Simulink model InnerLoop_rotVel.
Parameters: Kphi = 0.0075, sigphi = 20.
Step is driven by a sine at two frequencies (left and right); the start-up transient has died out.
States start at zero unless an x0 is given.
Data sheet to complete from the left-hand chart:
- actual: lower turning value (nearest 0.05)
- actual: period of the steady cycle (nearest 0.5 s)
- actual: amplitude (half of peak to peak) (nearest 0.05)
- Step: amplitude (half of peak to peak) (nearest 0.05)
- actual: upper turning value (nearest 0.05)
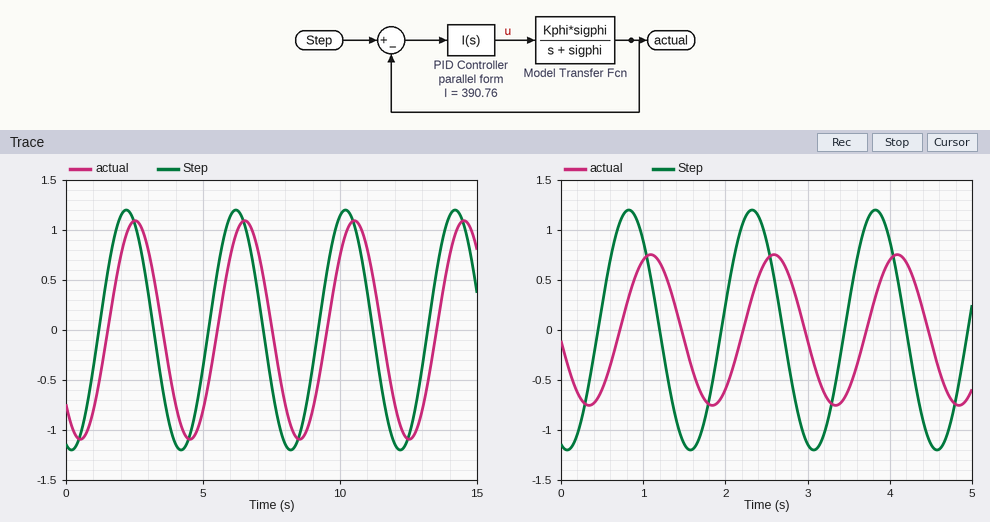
-1.10
4.0 s
1.10
1.20
1.10
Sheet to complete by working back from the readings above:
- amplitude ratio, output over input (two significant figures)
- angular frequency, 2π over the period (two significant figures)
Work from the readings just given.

0.92
1.6 rad/s
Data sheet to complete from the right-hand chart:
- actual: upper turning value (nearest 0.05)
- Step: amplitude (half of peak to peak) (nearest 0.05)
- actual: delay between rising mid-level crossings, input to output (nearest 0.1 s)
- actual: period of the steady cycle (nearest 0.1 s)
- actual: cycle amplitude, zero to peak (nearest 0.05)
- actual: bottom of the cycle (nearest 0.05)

0.75
1.20
0.3 s
1.5 s
0.75
-0.75
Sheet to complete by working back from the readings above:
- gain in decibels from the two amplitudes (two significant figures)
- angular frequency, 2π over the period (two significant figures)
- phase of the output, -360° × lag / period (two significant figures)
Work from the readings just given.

-4.1 dB
4.2 rad/s
-72°
